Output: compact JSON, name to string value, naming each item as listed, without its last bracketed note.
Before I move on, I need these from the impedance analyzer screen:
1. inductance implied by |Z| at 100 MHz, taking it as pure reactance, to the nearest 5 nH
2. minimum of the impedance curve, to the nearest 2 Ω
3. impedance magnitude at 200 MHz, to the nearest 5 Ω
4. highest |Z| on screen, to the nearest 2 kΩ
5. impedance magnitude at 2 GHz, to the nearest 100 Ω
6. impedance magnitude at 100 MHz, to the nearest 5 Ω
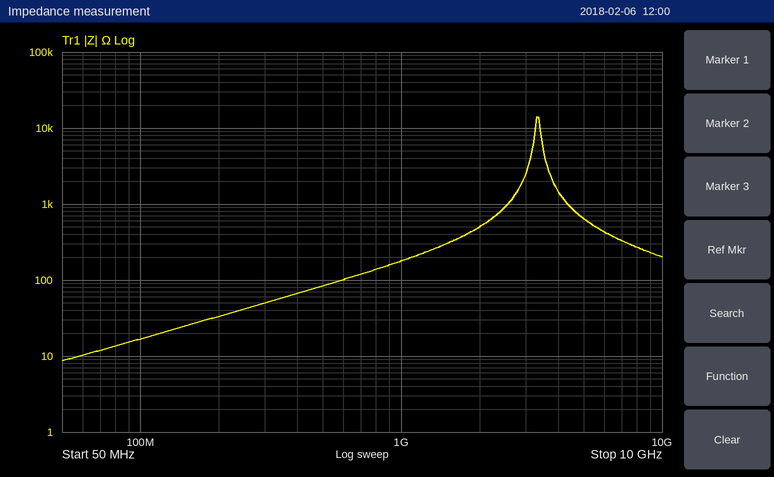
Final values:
{"inductance implied by |Z| at 100 MHz, taking it as pure reactance, to the nearest 5 nH": "25 nH", "minimum of the impedance curve, to the nearest 2 Ω": "8 Ω", "impedance magnitude at 200 MHz, to the nearest 5 Ω": "35 Ω", "highest |Z| on screen, to the nearest 2 kΩ": "14 kΩ", "impedance magnitude at 2 GHz, to the nearest 100 Ω": "500 Ω", "impedance magnitude at 100 MHz, to the nearest 5 Ω": "15 Ω"}
